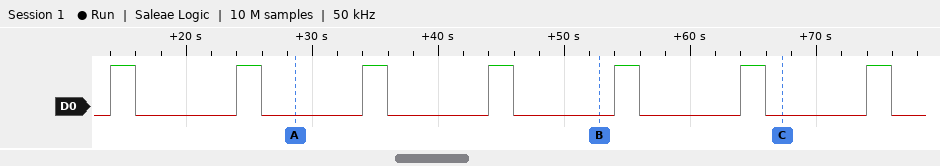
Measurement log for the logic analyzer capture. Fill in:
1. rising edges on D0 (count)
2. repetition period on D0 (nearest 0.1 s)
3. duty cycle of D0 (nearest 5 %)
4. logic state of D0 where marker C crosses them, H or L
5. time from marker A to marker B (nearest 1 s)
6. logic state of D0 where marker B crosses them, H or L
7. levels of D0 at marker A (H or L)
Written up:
7
10 s
20 %
D0=L
24 s
D0=L
D0=L
